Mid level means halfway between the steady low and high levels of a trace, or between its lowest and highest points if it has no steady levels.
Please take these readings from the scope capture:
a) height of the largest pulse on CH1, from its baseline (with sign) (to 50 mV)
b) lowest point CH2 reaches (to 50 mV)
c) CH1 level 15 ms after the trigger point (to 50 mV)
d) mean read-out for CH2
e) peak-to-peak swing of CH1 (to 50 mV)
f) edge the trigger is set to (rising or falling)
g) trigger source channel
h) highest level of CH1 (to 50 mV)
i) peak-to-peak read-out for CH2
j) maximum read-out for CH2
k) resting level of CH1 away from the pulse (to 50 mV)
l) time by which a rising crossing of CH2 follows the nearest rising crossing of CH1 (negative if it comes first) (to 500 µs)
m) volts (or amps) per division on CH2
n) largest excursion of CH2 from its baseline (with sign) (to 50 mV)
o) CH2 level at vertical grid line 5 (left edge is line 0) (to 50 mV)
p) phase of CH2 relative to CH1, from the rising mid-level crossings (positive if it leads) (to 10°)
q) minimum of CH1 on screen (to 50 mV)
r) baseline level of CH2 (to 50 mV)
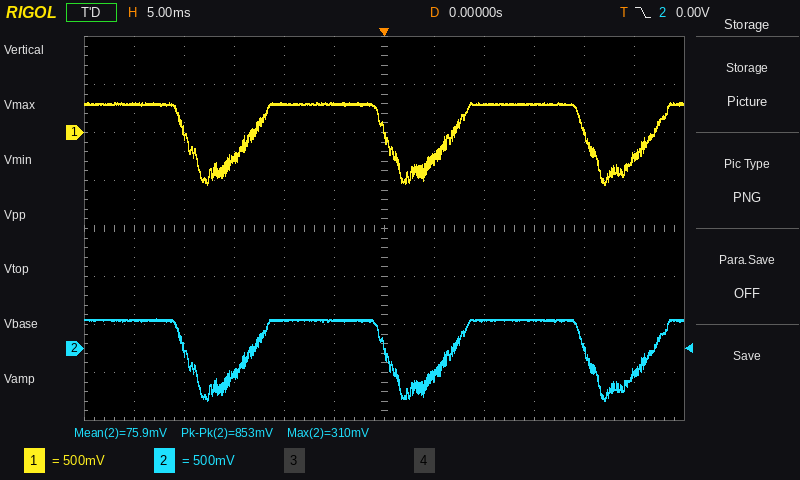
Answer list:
-850 mV
-550 mV
300 mV
75.9 mV
850 mV
falling
CH2
300 mV
853 mV
310 mV
300 mV
0.0 ms
500 mV
-850 mV
300 mV
0°
-550 mV
300 mV
